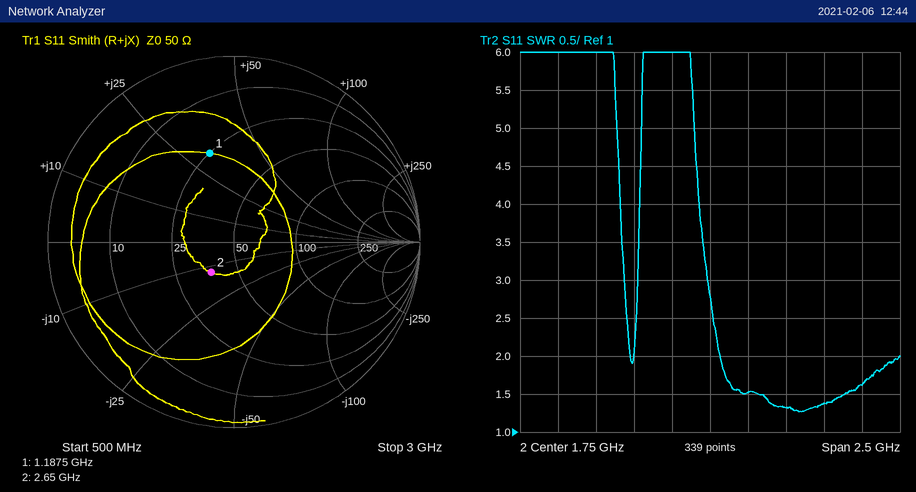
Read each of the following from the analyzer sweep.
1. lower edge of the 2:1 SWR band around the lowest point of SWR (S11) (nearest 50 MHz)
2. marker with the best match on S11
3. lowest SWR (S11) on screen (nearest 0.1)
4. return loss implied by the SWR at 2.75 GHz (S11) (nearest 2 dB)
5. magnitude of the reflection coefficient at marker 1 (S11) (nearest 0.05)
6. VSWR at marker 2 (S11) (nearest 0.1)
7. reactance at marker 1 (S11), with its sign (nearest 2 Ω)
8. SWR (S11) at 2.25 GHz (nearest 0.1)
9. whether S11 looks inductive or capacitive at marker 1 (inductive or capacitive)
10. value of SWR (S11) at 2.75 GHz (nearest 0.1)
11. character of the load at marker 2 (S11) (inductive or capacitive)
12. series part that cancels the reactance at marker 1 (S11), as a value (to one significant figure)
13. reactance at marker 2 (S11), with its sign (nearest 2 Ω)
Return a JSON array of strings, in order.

["1.80 GHz", "marker 2", "1.3", "12 dB", "0.50", "1.5", "+32 Ω", "1.3", "inductive", "1.6", "capacitive", "4 pF", "-12 Ω"]
